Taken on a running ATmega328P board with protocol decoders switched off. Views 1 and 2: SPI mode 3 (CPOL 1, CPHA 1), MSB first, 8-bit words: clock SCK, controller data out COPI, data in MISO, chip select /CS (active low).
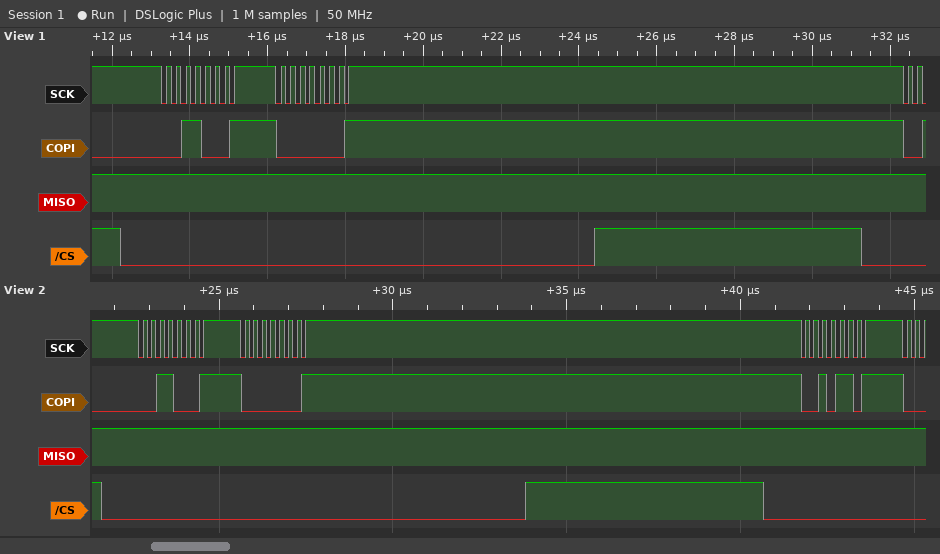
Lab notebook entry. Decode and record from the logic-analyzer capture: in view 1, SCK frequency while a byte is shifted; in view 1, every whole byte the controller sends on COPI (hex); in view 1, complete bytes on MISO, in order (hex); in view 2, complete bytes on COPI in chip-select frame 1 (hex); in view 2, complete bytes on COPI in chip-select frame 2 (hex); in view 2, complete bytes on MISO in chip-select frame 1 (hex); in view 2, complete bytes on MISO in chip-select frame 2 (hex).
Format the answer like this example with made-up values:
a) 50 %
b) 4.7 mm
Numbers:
a) 4 MHz
b) 31 01
c) FF FF
d) 0x31 0x01
e) 0x2D
f) 0xFF 0xFF
g) 0xFF
